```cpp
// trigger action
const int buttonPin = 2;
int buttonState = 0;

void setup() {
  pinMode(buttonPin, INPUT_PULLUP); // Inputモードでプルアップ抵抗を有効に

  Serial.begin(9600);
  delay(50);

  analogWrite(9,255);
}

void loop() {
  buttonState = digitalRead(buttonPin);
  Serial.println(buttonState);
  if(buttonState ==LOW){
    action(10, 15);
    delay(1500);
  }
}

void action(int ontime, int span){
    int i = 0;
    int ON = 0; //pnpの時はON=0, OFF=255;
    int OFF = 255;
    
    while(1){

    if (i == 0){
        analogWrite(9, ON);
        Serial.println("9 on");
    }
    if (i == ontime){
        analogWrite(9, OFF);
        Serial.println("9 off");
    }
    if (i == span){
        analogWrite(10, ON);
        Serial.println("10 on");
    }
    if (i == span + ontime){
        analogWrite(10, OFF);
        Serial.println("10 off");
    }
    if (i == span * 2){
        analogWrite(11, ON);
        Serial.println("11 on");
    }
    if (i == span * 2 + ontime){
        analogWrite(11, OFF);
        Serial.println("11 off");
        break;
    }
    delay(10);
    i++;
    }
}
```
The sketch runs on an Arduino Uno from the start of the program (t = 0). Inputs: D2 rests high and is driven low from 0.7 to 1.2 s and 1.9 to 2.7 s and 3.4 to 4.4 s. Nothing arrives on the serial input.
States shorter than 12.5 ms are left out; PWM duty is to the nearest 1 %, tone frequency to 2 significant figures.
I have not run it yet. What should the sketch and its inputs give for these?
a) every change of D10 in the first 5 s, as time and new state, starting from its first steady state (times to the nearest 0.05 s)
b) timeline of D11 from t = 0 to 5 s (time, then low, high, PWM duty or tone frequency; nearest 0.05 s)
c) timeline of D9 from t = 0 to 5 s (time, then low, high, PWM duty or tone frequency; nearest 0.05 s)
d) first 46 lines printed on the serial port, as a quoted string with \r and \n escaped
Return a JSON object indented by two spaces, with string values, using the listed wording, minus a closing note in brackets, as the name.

{
  "every change of D10 in the first 5 s, as time and new state, starting from its first steady state": "0.85 s low; 0.95 s high; 2.75 s low; 2.85 s high",
  "timeline of D11 from t = 0 to 5 s": "1 s low; 1.1 s high; 2.9 s low; 3 s high",
  "timeline of D9 from t = 0 to 5 s": "0.05 s high; 0.7 s low; 0.8 s high; 2.6 s low; 2.7 s high",
  "first 46 lines printed on the serial port, as a quoted string with \\r and \\n escaped": "\"1\\r\\n1\\r\\n1\\r\\n1\\r\\n1\\r\\n1\\r\\n1\\r\\n1\\r\\n1\\r\\n1\\r\\n1\\r\\n1\\r\\n1\\r\\n1\\r\\n1\\r\\n1\\r\\n1\\r\\n1\\r\\n1\\r\\n1\\r\\n1\\r\\n1\\r\\n1\\r\\n1\\r\\n1\\r\\n1\\r\\n1\\r\\n1\\r\\n1\\r\\n1\\r\\n1\\r\\n1\\r\\n1\\r\\n1\\r\\n1\\r\\n1\\r\\n1\\r\\n1\\r\\n1\\r\\n1\\r\\n1\\r\\n1\\r\\n1\\r\\n1\\r\\n1\\r\\n1\\r\\n\""
}
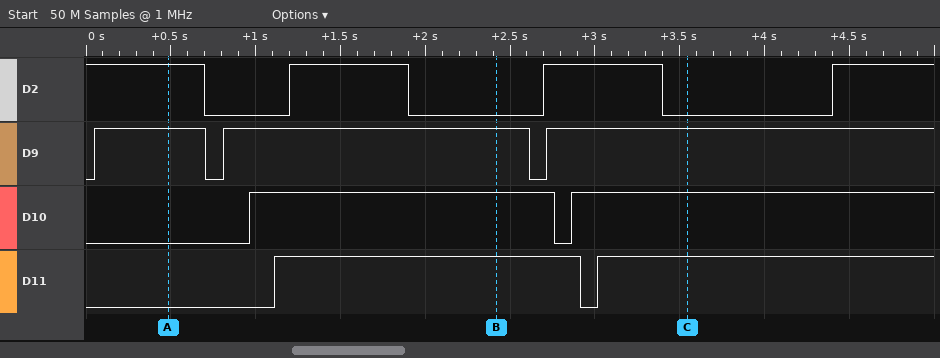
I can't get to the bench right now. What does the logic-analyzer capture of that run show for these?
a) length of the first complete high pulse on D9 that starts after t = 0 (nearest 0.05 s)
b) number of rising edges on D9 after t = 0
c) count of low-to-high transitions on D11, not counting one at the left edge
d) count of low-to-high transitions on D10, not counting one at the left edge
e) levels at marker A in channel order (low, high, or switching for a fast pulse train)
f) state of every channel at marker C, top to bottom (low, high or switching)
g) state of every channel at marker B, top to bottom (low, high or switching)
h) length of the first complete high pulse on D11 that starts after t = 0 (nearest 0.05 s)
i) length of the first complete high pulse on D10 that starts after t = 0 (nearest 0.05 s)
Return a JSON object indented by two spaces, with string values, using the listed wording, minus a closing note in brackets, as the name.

{
  "length of the first complete high pulse on D9 that starts after t = 0": "0.65 s",
  "number of rising edges on D9 after t = 0": "3",
  "count of low-to-high transitions on D11, not counting one at the left edge": "2",
  "count of low-to-high transitions on D10, not counting one at the left edge": "2",
  "levels at marker A in channel order": "D2 high, D9 high, D10 low, D11 low",
  "state of every channel at marker C, top to bottom": "D2 low, D9 high, D10 high, D11 high",
  "state of every channel at marker B, top to bottom": "D2 low, D9 high, D10 high, D11 high",
  "length of the first complete high pulse on D11 that starts after t = 0": "1.80 s",
  "length of the first complete high pulse on D10 that starts after t = 0": "1.80 s"
}
